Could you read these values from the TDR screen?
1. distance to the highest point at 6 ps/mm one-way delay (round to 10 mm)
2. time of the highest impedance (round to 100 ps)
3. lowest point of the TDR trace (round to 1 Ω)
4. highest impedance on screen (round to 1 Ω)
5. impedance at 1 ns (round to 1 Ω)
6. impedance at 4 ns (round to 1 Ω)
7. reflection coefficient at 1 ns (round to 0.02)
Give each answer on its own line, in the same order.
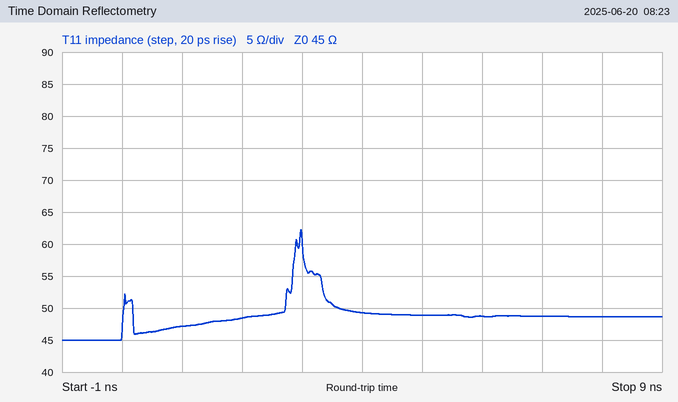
250 mm
3.0 ns
45 Ω
62 Ω
47 Ω
49 Ω
+0.02
